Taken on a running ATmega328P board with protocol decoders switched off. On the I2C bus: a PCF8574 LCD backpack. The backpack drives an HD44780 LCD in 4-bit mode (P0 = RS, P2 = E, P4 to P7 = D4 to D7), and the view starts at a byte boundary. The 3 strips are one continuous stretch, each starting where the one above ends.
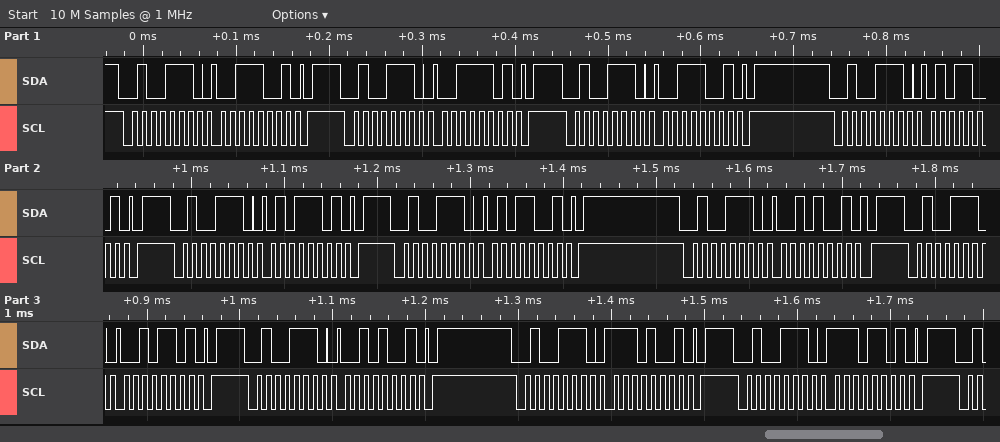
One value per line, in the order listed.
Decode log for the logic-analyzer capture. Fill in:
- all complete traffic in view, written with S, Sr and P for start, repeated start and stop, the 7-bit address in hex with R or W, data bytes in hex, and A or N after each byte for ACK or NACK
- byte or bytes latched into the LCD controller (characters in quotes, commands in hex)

S 27W A 39 A P S 27W A 3D A P S 27W A 39 A P S 27W A 59 A P S 27W A 5D A P S 27W A 59 A P S 27W A 29 A P S 27W A 2D A P S 27W A 29 A P S 27W A E9 A P S 27W A ED A P
'5'
